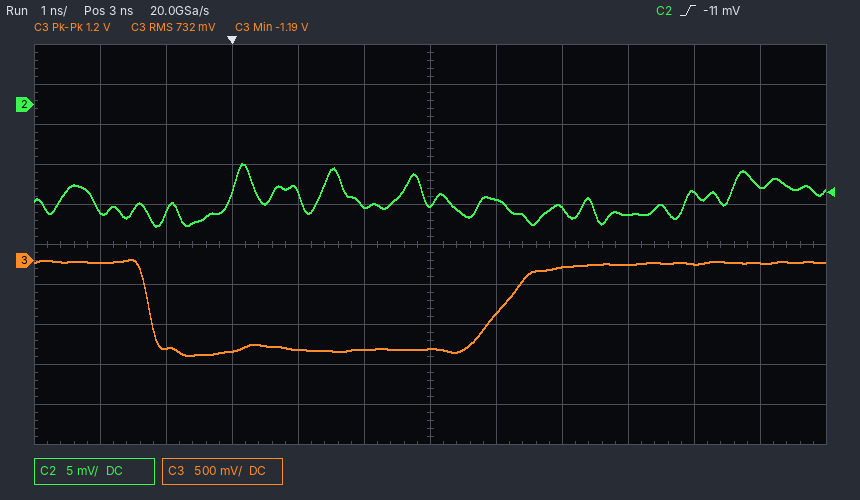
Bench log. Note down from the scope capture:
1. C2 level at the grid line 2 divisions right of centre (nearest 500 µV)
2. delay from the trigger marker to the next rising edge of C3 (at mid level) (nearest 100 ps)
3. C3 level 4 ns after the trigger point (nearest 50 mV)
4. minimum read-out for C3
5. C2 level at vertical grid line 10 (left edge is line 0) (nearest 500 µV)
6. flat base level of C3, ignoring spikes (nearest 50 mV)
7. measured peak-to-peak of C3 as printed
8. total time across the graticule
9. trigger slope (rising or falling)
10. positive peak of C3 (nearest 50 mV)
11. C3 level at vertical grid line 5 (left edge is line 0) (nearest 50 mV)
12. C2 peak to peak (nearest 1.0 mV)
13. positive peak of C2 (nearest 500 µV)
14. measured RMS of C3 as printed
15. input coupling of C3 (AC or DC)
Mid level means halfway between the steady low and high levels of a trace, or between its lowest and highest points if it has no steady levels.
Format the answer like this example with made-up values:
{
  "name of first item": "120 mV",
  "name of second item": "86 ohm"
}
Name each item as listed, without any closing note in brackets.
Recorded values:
{
  "C2 level at the grid line 2 divisions right of centre": "-13.0 mV",
  "delay from the trigger marker to the next rising edge of C3 (at mid level)": "4.1 ns",
  "C3 level 4 ns after the trigger point": "-650 mV",
  "minimum read-out for C3": "-1.19 V",
  "C2 level at vertical grid line 10 (left edge is line 0)": "-11.0 mV",
  "flat base level of C3, ignoring spikes": "-1.10 V",
  "measured peak-to-peak of C3 as printed": "1.2 V",
  "total time across the graticule": "12 ns",
  "trigger slope": "rising",
  "positive peak of C3": "0 mV",
  "C3 level at vertical grid line 5 (left edge is line 0)": "-1.10 V",
  "C2 peak to peak": "8.0 mV",
  "positive peak of C2": "-7.5 mV",
  "measured RMS of C3 as printed": "732 mV",
  "input coupling of C3": "DC"
}
